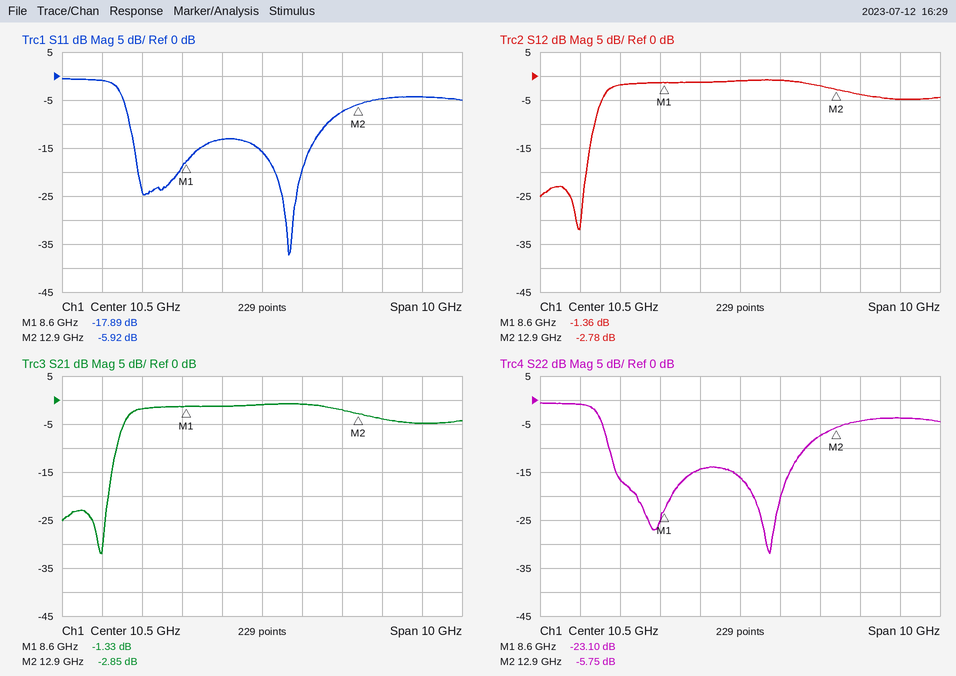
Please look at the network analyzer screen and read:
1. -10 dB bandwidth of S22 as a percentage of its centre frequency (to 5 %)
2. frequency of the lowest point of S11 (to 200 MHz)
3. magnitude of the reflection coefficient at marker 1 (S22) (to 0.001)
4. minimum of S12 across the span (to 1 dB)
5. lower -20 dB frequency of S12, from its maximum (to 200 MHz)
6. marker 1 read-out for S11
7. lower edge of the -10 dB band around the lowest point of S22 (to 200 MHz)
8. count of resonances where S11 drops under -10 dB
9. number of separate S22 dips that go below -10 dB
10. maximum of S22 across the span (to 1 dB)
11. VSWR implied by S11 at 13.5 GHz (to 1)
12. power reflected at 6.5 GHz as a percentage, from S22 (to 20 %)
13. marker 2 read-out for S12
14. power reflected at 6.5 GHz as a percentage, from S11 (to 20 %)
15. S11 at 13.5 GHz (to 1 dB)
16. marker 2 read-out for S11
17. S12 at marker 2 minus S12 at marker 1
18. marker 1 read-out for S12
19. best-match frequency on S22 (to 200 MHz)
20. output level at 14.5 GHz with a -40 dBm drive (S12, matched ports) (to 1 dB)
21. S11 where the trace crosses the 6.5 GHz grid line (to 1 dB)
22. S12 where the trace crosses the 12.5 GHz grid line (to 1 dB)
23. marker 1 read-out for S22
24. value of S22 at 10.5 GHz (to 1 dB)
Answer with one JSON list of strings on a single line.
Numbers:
["50 %", "11.2 GHz", "0.070", "-32 dB", "6.6 GHz", "-17.89 dB", "7.2 GHz", "2", "2", "-1 dB", "4", "80 %", "-2.78 dB", "80 %", "-5 dB", "-5.92 dB", "-1.42 dB", "-1.36 dB", "11.2 GHz", "-45 dBm", "-1 dB", "-2 dB", "-23.10 dB", "-16 dB"]
